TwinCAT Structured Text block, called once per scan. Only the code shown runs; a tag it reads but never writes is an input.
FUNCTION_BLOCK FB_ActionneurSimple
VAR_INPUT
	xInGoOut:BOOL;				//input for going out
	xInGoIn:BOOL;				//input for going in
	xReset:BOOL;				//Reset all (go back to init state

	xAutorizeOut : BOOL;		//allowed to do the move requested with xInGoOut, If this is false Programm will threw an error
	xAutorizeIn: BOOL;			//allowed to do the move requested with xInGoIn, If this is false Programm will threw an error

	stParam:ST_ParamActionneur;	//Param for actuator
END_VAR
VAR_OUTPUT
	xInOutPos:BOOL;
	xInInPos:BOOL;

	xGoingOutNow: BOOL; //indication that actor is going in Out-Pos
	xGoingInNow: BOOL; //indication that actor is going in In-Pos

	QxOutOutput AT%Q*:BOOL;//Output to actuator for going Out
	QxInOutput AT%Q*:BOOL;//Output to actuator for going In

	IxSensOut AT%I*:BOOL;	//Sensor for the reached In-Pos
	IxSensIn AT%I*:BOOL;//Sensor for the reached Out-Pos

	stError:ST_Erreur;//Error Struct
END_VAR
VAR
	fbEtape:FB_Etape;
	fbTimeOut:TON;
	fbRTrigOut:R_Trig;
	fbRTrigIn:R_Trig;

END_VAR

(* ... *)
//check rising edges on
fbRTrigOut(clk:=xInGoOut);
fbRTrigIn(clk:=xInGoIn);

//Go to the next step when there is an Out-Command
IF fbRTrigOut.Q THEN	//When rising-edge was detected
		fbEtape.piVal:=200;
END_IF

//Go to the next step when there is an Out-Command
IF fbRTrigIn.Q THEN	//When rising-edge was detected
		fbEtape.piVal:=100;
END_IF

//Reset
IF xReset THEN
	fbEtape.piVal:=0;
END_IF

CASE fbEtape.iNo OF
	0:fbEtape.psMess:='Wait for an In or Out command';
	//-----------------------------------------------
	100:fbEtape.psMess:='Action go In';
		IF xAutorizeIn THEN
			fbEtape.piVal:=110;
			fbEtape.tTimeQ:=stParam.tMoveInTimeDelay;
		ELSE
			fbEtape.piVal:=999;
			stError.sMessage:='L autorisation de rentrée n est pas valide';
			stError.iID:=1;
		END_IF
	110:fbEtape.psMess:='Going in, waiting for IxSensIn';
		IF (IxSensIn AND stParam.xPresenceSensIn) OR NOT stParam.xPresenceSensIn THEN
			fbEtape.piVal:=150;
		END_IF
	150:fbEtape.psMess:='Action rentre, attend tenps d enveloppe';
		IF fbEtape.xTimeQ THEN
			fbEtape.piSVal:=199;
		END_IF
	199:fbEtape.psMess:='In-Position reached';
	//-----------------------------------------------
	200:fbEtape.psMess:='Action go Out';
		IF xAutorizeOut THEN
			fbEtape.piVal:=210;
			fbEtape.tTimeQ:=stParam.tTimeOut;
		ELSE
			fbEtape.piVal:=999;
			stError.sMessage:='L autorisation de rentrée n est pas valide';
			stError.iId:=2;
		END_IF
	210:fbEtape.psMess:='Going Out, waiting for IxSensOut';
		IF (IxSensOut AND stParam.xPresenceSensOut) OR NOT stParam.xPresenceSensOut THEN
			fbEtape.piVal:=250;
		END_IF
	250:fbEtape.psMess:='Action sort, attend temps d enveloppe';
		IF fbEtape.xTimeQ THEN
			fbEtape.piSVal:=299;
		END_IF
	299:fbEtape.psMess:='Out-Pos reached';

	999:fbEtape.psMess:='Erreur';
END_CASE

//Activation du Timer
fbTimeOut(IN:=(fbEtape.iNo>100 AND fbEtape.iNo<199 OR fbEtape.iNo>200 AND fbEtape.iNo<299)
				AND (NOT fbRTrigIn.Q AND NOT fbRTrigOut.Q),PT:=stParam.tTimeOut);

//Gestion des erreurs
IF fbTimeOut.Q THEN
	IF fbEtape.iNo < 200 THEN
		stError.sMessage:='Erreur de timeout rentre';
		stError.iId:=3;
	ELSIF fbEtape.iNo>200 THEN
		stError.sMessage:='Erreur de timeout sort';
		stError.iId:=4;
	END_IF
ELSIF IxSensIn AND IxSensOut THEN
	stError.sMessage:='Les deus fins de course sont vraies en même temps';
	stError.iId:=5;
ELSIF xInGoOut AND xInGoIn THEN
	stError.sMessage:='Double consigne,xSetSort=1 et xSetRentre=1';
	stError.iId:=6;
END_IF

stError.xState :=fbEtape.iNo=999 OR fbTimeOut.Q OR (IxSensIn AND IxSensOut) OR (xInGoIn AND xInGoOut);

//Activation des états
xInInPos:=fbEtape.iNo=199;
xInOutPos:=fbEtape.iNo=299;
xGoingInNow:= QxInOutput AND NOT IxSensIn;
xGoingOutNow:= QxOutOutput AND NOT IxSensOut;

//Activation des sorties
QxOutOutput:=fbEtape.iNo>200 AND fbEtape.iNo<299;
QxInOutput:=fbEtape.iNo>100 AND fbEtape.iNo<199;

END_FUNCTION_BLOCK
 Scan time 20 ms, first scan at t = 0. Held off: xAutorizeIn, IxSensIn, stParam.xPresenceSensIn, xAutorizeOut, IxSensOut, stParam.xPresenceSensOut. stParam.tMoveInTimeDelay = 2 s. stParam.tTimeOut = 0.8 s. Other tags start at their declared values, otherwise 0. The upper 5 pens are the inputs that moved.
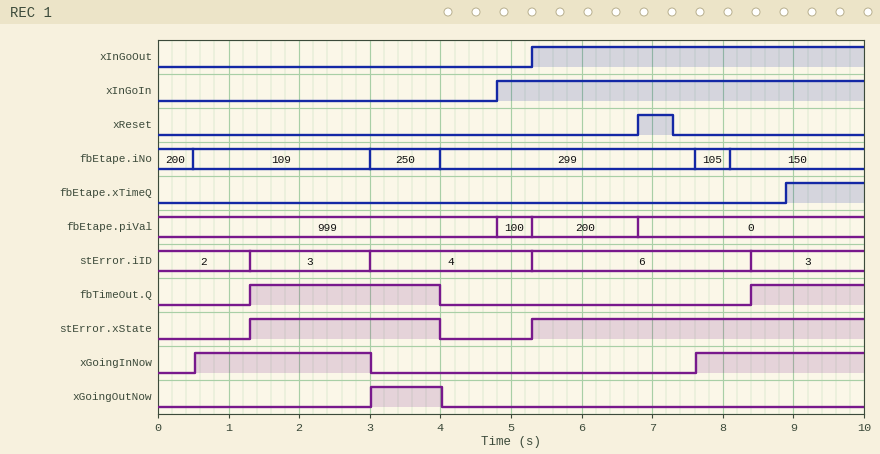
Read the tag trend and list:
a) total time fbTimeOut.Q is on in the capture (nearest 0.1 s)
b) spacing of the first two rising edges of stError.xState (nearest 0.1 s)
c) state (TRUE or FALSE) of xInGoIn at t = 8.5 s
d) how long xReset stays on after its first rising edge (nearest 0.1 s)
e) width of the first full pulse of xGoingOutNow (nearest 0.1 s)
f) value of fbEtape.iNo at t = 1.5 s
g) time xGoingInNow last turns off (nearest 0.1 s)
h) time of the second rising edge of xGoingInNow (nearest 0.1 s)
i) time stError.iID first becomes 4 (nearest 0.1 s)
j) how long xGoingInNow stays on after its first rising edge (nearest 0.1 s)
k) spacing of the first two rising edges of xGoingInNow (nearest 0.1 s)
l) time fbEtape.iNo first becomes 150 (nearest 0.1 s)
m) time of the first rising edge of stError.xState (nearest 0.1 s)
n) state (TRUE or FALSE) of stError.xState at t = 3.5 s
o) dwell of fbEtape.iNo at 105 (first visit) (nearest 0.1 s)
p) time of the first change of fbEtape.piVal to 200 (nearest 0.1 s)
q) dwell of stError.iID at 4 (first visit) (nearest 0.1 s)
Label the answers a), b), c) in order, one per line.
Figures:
a) 4.3 s
b) 4.0 s
c) TRUE
d) 0.5 s
e) 1.0 s
f) 109
g) 3.0 s
h) 7.6 s
i) 3.0 s
j) 2.5 s
k) 7.1 s
l) 8.1 s
m) 1.3 s
n) TRUE
o) 0.5 s
p) 5.3 s
q) 2.3 s
